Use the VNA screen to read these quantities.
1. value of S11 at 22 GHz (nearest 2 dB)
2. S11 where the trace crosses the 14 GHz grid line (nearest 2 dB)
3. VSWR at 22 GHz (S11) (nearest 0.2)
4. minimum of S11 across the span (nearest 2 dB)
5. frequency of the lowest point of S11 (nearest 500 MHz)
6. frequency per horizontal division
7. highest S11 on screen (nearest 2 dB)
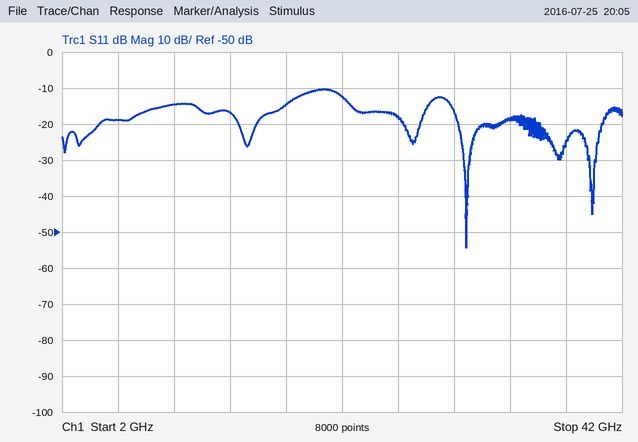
-12 dB
-16 dB
1.6
-54 dB
31.0 GHz
4 GHz
-10 dB
